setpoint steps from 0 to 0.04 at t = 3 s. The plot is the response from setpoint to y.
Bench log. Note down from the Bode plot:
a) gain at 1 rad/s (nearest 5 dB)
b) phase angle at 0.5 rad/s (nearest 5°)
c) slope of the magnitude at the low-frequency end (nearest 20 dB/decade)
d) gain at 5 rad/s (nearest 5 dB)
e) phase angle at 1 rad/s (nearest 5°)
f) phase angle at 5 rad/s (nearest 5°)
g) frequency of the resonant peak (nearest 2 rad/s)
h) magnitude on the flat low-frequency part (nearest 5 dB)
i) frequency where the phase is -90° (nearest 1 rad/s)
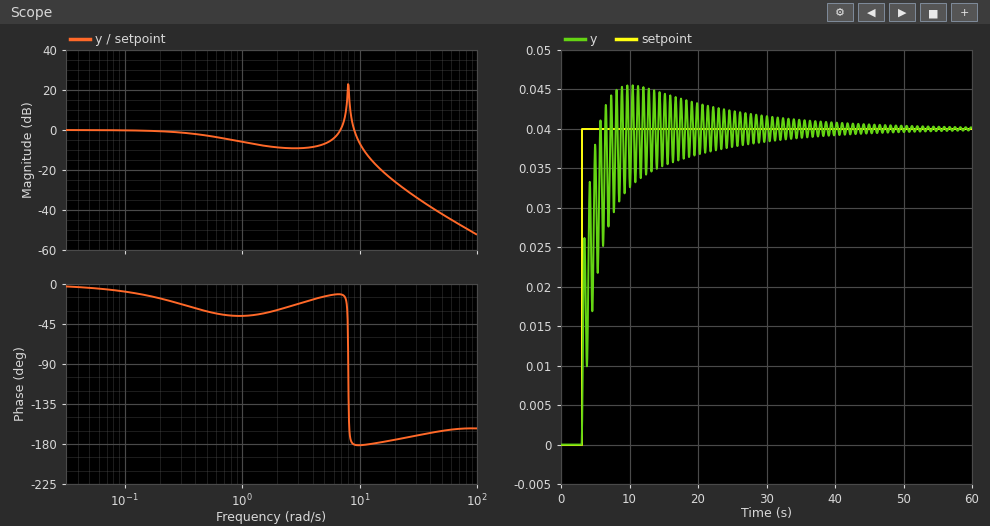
-5 dB
-30°
0 dB/decade
-5 dB
-35°
-15°
8 rad/s
0 dB
8 rad/s
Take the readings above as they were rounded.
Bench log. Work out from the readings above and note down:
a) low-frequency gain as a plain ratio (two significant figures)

1.0
